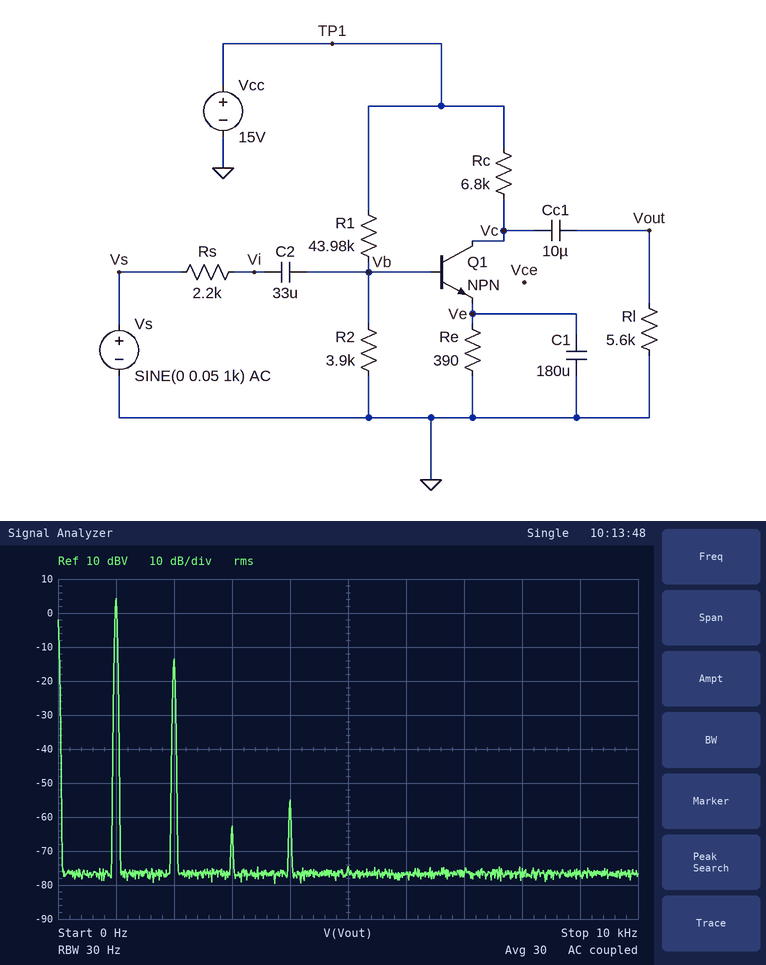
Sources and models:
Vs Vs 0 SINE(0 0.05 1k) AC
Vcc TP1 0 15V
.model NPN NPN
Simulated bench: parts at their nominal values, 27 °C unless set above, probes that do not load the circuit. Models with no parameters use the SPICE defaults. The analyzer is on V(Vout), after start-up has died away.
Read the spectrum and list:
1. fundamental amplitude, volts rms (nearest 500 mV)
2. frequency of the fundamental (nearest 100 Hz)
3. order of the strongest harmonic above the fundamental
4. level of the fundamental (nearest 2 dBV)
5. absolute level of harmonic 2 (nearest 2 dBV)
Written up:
1.5 V
1.0 kHz
2
4 dBV
-14 dBV
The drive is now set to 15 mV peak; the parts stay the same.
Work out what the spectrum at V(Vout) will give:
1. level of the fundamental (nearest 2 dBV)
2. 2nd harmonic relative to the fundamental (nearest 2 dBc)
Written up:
-6 dBV
-28 dBc
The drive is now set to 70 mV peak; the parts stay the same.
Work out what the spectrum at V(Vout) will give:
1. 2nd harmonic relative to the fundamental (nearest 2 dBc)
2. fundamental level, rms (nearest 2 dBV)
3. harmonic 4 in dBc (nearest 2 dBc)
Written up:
-14 dBc
6 dBV
-50 dBc
